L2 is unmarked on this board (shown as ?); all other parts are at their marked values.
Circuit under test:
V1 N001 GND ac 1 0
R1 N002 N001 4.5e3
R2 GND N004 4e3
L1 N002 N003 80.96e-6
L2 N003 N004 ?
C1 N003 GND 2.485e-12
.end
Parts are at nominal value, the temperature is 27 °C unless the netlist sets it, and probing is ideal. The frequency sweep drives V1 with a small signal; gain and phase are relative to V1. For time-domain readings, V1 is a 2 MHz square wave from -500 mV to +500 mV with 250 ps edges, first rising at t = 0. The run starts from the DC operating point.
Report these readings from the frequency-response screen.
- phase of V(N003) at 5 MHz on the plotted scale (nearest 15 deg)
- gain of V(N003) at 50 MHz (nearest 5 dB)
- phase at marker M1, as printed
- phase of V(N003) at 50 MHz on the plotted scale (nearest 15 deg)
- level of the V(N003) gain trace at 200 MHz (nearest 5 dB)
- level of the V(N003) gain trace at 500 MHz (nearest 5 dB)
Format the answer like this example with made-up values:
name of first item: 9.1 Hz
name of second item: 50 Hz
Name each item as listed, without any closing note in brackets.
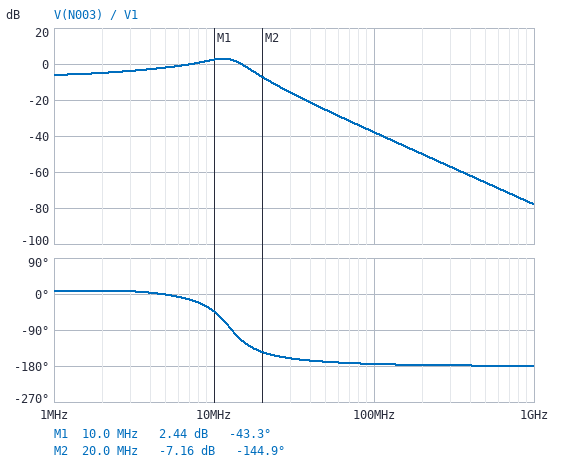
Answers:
phase of V(N003) at 5 MHz on the plotted scale: 0 deg
gain of V(N003) at 50 MHz: -25 dB
phase at marker M1, as printed: -43.3 deg
phase of V(N003) at 50 MHz on the plotted scale: -165 deg
level of the V(N003) gain trace at 200 MHz: -50 dB
level of the V(N003) gain trace at 500 MHz: -65 dB
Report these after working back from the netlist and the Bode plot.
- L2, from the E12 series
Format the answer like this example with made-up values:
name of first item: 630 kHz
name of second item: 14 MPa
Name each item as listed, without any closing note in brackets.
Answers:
L2, from the E12 series: 270 µH
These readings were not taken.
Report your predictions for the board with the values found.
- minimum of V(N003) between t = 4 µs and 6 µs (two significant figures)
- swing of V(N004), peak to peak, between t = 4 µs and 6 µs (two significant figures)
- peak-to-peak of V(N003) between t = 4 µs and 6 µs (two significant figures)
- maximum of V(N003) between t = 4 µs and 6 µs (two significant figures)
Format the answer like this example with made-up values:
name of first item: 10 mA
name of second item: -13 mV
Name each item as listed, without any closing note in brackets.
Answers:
minimum of V(N003) between t = 4 µs and 6 µs: -700 mV
swing of V(N004), peak to peak, between t = 4 µs and 6 µs: 470 mV
peak-to-peak of V(N003) between t = 4 µs and 6 µs: 1.4 V
maximum of V(N003) between t = 4 µs and 6 µs: 700 mV
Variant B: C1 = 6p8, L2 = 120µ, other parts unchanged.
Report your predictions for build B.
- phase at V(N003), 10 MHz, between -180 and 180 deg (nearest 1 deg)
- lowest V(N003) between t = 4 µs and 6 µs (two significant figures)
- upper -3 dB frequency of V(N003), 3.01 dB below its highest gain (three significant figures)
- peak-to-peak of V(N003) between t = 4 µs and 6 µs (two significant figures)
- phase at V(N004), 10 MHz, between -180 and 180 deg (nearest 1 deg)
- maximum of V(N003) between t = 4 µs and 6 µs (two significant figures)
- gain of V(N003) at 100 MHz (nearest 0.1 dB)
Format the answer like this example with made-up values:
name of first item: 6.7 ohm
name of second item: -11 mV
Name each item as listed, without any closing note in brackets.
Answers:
phase at V(N003), 10 MHz, between -180 and 180 deg: -103 deg
lowest V(N003) between t = 4 µs and 6 µs: -400 mV
upper -3 dB frequency of V(N003), 3.01 dB below its highest gain: 10.5 MHz
peak-to-peak of V(N003) between t = 4 µs and 6 µs: 800 mV
phase at V(N004), 10 MHz, between -180 and 180 deg: -165 deg
maximum of V(N003) between t = 4 µs and 6 µs: 400 mV
gain of V(N003) at 100 MHz: -46.7 dB
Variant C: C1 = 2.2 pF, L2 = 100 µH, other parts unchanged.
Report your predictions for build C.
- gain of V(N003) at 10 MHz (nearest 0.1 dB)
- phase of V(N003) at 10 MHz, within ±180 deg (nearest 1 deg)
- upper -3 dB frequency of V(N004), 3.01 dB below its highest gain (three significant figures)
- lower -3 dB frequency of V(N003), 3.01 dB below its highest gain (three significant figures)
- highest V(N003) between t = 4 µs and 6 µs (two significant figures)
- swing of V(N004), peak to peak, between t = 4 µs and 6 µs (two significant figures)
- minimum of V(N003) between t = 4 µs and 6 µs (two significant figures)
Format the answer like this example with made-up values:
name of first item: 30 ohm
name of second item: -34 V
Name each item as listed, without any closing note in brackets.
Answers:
gain of V(N003) at 10 MHz: -2.2 dB
phase of V(N003) at 10 MHz, within ±180 deg: -22 deg
upper -3 dB frequency of V(N004), 3.01 dB below its highest gain: 17.5 MHz
lower -3 dB frequency of V(N003), 3.01 dB below its highest gain: 10.6 MHz
highest V(N003) between t = 4 µs and 6 µs: 510 mV
swing of V(N004), peak to peak, between t = 4 µs and 6 µs: 520 mV
minimum of V(N003) between t = 4 µs and 6 µs: -510 mV
